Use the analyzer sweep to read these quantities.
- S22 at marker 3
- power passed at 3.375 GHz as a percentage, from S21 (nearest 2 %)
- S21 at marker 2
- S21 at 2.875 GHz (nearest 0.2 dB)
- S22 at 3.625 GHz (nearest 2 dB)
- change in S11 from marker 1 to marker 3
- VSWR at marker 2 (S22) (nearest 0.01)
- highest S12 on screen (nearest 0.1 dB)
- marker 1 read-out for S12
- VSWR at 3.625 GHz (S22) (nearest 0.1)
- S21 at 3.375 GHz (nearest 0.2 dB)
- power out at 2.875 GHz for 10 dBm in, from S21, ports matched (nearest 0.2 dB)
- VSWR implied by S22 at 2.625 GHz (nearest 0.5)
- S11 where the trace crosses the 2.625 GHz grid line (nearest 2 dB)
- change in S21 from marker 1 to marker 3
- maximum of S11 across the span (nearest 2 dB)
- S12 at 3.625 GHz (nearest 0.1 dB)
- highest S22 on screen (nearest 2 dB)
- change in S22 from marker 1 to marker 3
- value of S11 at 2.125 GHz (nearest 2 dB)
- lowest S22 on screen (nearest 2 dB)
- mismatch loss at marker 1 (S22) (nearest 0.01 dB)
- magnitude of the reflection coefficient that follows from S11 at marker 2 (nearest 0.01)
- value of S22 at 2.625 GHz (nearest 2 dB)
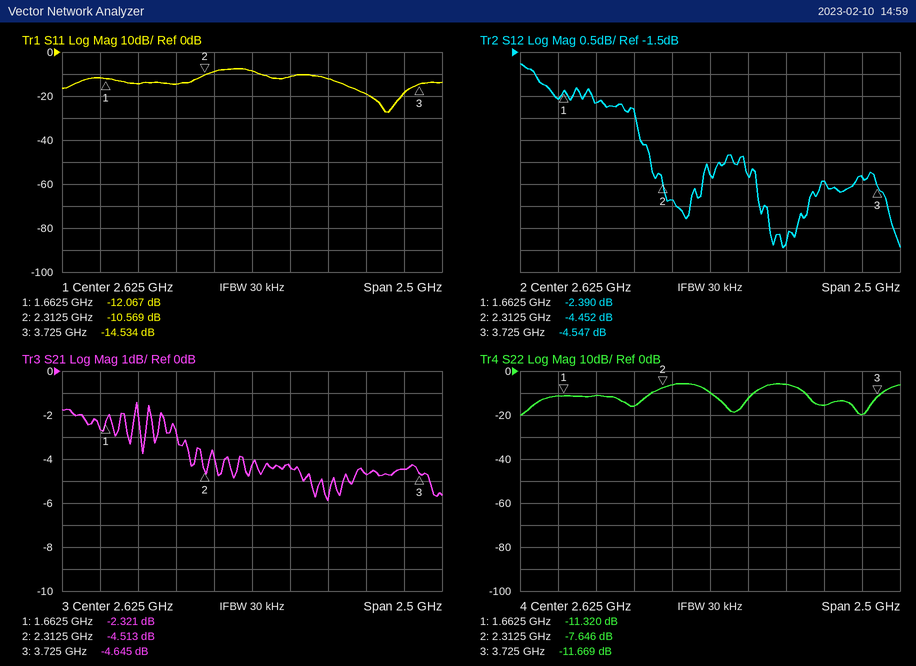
-11.669 dB
34 %
-4.513 dB
-4.4 dB
-20 dB
-2.467 dB
2.42
-1.8 dB
-2.390 dB
1.2
-4.6 dB
5.6 dBm
2.0
-8 dB
-2.324 dB
-8 dB
-4.3 dB
-6 dB
-0.349 dB
-14 dB
-20 dB
0.33 dB
0.30
-10 dB
